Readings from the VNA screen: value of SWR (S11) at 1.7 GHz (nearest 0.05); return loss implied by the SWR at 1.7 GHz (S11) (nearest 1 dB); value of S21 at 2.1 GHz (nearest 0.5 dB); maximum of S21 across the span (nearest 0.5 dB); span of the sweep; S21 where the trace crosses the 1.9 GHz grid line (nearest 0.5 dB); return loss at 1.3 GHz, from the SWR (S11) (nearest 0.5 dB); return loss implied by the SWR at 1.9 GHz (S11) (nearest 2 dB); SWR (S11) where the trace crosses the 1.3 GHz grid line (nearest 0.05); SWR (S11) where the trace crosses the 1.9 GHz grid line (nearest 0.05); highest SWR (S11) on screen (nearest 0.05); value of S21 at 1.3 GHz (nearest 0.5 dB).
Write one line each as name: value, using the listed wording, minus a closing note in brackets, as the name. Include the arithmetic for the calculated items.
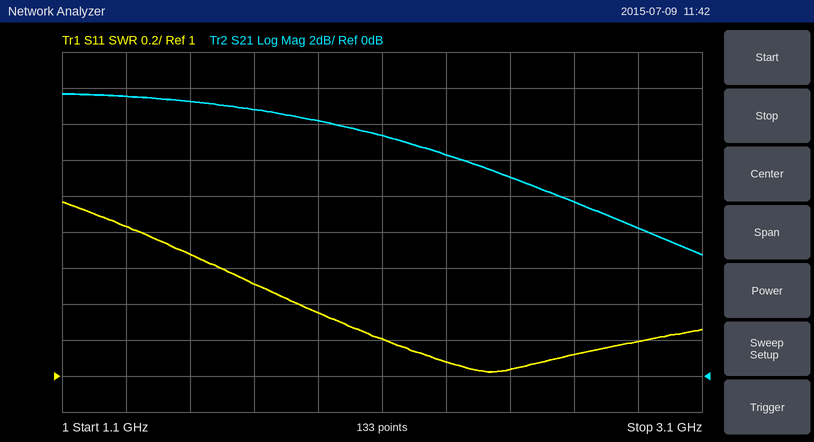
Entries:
value of SWR (S11) at 1.7 GHz: 1.50
return loss implied by the SWR at 1.7 GHz (S11): −20 log10((1.5 − 1)/(1.5 + 1)) ≈ 14 dB
value of S21 at 2.1 GHz: 13.5 dB
maximum of S21 across the span: 15.5 dB
span of the sweep: 2 GHz
S21 where the trace crosses the 1.9 GHz grid line: 14.0 dB
return loss at 1.3 GHz, from the SWR (S11): −20 log10((1.85 − 1)/(1.85 + 1)) ≈ 10.5 dB
return loss implied by the SWR at 1.9 GHz (S11): −20 log10((1.35 − 1)/(1.35 + 1)) ≈ 16 dB
SWR (S11) where the trace crosses the 1.3 GHz grid line: 1.85
SWR (S11) where the trace crosses the 1.9 GHz grid line: 1.35
highest SWR (S11) on screen: 1.95
value of S21 at 1.3 GHz: 15.5 dB
